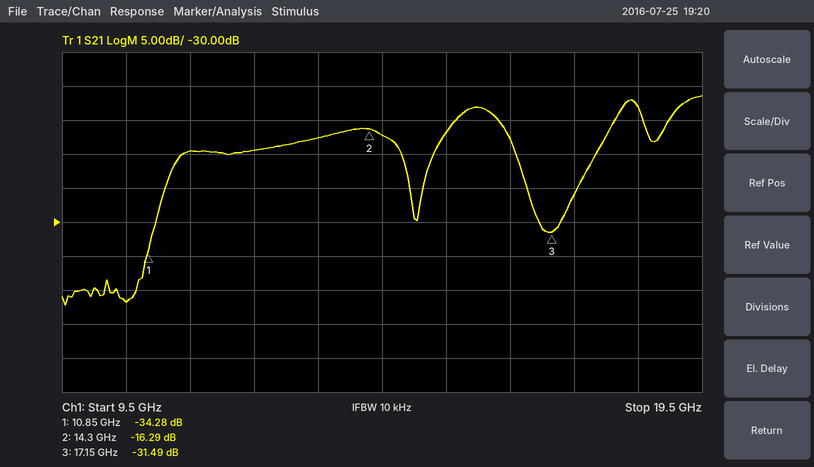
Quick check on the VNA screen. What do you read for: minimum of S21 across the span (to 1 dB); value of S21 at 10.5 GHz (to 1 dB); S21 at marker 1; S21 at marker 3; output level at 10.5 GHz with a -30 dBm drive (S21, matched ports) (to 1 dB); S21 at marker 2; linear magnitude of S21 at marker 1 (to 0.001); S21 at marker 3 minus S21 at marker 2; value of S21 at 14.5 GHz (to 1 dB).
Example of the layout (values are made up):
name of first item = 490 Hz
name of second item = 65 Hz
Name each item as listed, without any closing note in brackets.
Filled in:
minimum of S21 across the span = -42 dB
value of S21 at 10.5 GHz = -42 dB
S21 at marker 1 = -34.28 dB
S21 at marker 3 = -31.49 dB
output level at 10.5 GHz with a -30 dBm drive (S21, matched ports) = -72 dBm
S21 at marker 2 = -16.29 dB
linear magnitude of S21 at marker 1 = 0.019
S21 at marker 3 minus S21 at marker 2 = -15.20 dB
value of S21 at 14.5 GHz = -17 dB
